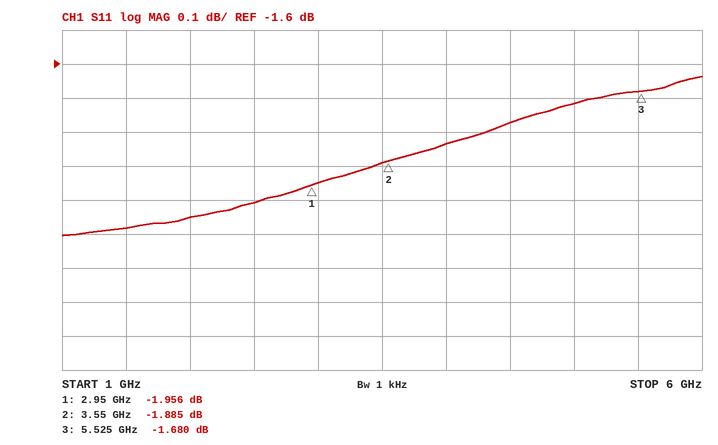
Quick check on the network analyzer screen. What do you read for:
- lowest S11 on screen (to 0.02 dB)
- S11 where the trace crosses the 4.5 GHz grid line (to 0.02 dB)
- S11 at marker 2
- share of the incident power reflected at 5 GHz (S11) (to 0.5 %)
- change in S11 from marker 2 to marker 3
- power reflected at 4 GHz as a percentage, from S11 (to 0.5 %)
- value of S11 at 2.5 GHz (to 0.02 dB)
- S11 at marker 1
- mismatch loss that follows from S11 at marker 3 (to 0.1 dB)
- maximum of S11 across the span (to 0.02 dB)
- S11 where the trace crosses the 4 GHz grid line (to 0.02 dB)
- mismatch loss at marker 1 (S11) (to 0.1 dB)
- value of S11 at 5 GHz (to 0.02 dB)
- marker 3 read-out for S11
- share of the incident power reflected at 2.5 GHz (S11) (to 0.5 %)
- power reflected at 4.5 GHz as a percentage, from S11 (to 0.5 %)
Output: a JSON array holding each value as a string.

["-2.10 dB", "-1.78 dB", "-1.885 dB", "67.5 %", "0.205 dB", "65.5 %", "-2.00 dB", "-1.956 dB", "4.9 dB", "-1.64 dB", "-1.84 dB", "4.4 dB", "-1.72 dB", "-1.680 dB", "63.0 %", "66.5 %"]
